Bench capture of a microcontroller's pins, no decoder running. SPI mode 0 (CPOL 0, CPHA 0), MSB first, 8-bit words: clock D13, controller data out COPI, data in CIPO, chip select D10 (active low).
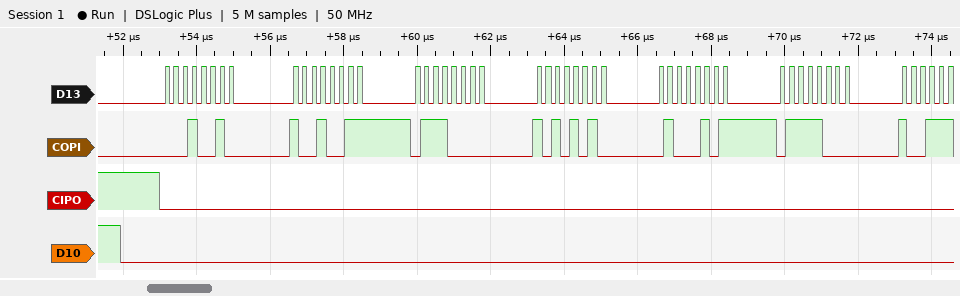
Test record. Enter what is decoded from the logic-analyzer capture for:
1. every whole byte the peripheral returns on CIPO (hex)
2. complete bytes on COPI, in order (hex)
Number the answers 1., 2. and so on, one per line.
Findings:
1. 00 00 00 00 00 00
2. 12 93 70 AA 45 78
